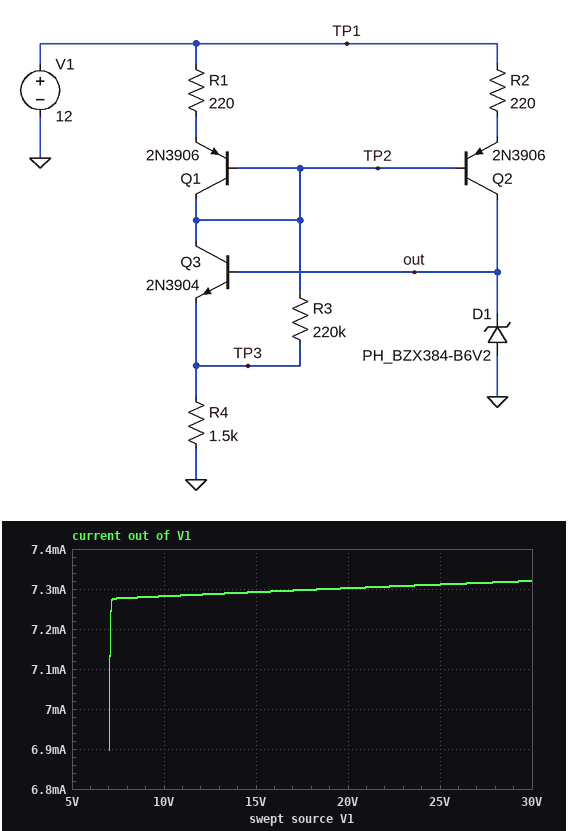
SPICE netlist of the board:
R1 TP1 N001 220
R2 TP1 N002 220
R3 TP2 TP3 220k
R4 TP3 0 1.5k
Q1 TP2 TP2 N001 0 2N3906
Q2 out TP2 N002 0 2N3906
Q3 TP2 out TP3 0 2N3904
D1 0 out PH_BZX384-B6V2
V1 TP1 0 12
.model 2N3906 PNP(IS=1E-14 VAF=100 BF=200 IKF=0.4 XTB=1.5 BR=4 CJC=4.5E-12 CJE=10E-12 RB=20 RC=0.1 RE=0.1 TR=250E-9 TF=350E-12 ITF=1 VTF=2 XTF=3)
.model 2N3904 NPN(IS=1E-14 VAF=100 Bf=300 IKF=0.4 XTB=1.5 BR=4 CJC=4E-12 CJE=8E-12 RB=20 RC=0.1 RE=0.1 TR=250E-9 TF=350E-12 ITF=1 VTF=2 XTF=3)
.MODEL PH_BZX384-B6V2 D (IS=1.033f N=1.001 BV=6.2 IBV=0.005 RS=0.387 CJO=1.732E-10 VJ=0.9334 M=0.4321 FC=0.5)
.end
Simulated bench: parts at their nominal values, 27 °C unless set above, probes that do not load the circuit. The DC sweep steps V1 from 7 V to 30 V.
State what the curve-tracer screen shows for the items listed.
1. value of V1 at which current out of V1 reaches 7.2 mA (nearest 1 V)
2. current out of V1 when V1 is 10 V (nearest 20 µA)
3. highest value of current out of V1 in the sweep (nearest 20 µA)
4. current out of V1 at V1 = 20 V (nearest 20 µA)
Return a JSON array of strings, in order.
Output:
["7 V", "7.28 mA", "7.32 mA", "7.30 mA"]
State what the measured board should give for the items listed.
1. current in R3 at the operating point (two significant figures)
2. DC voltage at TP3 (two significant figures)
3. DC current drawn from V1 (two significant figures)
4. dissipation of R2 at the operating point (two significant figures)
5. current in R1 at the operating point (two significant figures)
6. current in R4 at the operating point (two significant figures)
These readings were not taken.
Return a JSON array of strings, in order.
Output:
["23 µA", "5.5 V", "7.3 mA", "2.9 mW", "3.6 mA", "3.7 mA"]
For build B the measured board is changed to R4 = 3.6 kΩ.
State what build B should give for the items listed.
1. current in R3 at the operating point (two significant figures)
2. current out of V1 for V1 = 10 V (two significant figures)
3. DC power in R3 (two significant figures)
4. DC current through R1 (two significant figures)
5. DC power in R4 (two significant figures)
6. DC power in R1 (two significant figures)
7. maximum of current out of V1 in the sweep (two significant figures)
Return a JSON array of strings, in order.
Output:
["25 µA", "3.0 mA", "140 µW", "1.5 mA", "8.4 mW", "510 µW", "3.1 mA"]
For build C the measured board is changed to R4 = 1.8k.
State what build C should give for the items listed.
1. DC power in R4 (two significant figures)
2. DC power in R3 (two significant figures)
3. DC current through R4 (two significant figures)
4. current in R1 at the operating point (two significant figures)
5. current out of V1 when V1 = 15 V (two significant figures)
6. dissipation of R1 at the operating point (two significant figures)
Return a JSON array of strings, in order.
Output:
["17 mW", "120 µW", "3.1 mA", "3.0 mA", "6.1 mA", "2.0 mW"]
